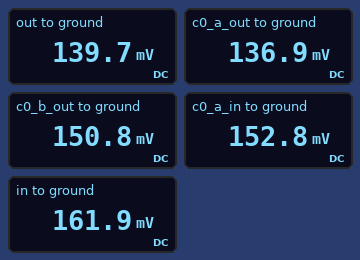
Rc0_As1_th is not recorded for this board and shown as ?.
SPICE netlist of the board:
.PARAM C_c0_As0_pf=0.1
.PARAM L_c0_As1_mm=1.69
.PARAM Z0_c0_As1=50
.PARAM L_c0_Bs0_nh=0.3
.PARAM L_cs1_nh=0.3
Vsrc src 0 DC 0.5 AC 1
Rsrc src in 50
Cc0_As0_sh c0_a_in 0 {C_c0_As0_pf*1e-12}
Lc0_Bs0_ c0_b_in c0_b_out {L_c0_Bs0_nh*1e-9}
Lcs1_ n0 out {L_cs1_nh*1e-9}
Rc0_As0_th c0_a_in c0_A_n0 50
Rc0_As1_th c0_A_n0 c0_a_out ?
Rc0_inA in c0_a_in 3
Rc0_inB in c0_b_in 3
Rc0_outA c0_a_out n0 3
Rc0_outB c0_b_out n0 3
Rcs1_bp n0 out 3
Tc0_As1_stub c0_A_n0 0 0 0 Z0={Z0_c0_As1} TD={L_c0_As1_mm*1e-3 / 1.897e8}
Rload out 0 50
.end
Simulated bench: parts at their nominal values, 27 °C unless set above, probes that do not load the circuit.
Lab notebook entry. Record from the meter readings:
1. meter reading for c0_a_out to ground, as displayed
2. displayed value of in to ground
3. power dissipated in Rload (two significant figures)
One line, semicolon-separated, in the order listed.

136.9 mV; 161.9 mV; 390 µW
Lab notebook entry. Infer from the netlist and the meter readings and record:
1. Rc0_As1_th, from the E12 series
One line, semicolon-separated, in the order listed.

150 Ω
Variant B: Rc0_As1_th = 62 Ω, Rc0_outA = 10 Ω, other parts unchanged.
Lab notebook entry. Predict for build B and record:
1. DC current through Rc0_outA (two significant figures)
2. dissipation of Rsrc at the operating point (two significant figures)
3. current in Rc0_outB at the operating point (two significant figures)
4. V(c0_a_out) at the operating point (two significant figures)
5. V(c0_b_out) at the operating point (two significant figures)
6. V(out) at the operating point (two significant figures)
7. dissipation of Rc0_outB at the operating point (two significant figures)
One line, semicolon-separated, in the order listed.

1.7 mA; 2.5 mW; 4.2 mA; 110 mV; 140 mV; 120 mV; 53 µW
